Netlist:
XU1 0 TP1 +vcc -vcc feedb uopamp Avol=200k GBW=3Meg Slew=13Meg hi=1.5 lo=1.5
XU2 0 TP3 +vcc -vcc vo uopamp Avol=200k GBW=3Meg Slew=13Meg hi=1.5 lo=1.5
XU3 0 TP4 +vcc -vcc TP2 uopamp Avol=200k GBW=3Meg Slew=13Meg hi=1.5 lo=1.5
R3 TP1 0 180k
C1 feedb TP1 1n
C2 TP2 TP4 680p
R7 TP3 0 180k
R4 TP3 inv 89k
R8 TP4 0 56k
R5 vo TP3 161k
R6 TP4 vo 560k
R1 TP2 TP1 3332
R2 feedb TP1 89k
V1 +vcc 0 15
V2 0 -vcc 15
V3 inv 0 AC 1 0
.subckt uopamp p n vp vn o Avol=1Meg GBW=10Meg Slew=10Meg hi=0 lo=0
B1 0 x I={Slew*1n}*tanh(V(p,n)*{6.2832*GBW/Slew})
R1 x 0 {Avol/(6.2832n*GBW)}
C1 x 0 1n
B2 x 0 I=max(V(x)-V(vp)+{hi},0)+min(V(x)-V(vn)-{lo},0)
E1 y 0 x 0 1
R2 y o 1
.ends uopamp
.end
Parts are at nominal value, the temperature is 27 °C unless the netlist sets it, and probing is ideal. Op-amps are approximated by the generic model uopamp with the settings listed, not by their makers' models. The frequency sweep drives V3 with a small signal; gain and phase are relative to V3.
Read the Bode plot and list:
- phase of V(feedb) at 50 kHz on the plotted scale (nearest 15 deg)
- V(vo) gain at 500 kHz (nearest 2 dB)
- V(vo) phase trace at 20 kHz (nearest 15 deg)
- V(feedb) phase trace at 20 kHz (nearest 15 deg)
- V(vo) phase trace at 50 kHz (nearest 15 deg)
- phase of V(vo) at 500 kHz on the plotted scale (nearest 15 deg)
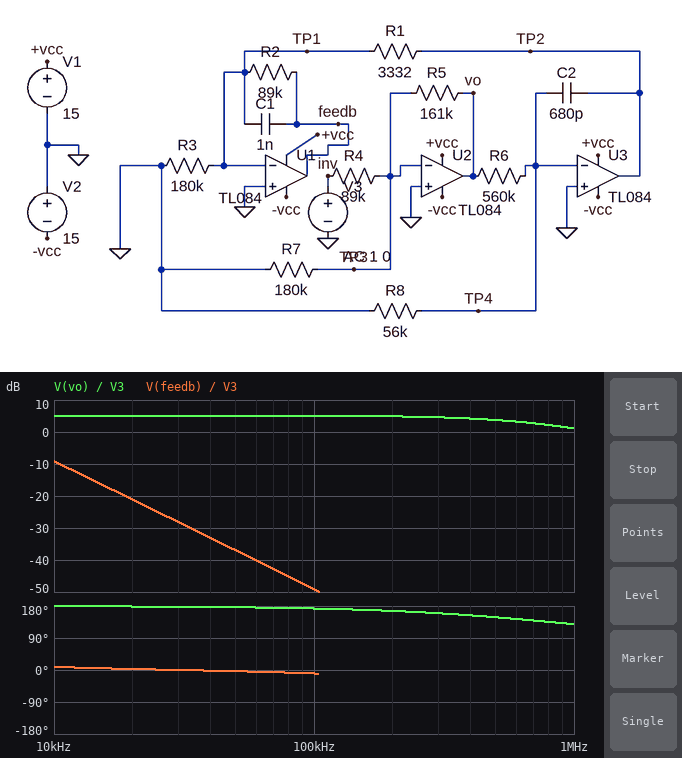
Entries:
0 deg
4 dB
180 deg
0 deg
180 deg
150 deg
